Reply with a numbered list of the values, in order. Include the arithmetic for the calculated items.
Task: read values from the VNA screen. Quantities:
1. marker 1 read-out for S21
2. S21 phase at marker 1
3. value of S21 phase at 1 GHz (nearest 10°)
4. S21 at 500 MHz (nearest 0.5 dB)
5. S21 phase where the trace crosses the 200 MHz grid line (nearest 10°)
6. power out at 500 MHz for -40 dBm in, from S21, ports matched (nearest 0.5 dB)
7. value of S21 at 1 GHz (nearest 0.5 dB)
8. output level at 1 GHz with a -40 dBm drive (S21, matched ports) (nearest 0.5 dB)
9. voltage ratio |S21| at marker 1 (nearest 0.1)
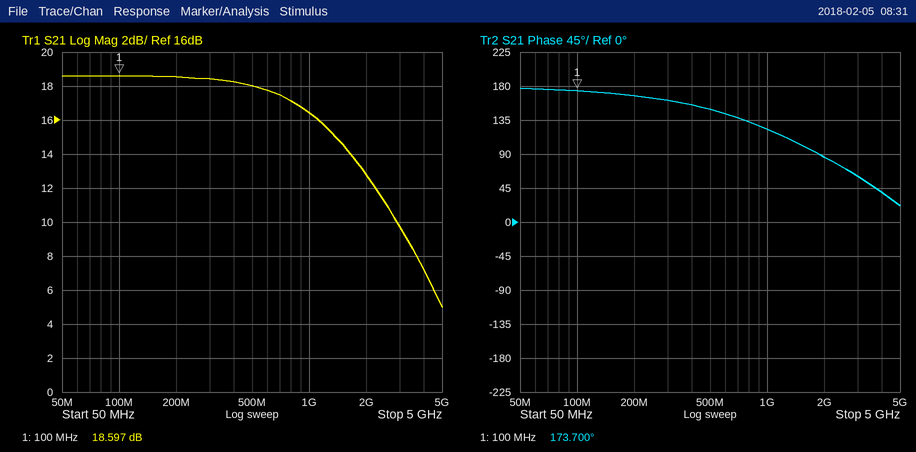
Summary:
1. 18.597 dB
2. 173.700°
3. 120°
4. 18.0 dB
5. 170°
6. -40 dBm + (18.0 dB) = -22.0 dBm
7. 16.5 dB
8. -40 dBm + (16.5 dB) = -23.5 dBm
9. 10^(18.597/20) ≈ 8.5
